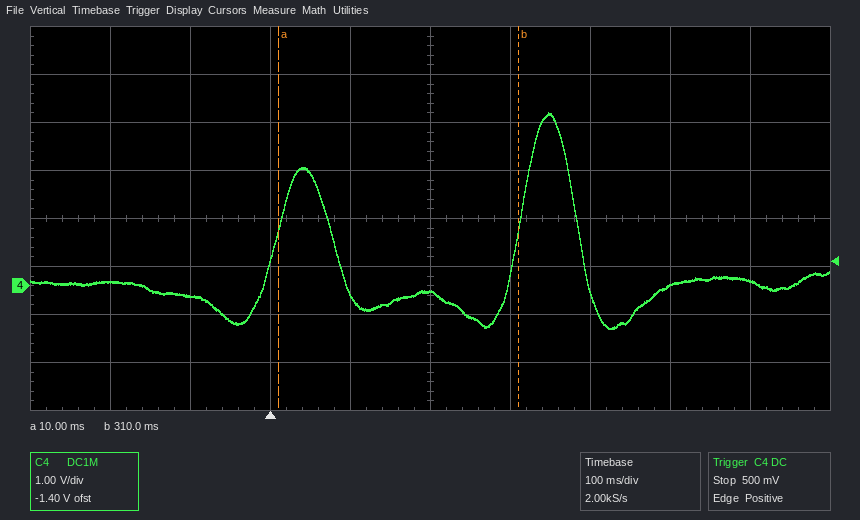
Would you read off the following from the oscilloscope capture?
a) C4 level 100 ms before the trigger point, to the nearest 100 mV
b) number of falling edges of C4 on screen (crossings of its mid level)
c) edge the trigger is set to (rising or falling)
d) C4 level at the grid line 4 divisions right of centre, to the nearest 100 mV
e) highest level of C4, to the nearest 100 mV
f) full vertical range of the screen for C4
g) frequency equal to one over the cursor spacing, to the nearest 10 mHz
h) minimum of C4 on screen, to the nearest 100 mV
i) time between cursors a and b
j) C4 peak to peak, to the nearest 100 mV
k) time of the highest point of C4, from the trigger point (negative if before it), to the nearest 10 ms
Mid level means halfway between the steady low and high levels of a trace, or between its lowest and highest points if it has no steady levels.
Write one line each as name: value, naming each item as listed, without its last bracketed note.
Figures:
C4 level 100 ms before the trigger point, to the nearest 100 mV: -200 mV
number of falling edges of C4 on screen: 2
edge the trigger is set to: rising
C4 level at the grid line 4 divisions right of centre, to the nearest 100 mV: 100 mV
highest level of C4, to the nearest 100 mV: 3.6 V
full vertical range of the screen for C4: 8 V
frequency equal to one over the cursor spacing, to the nearest 10 mHz: 3.33 Hz
minimum of C4 on screen, to the nearest 100 mV: -900 mV
time between cursors a and b: 300 ms
C4 peak to peak, to the nearest 100 mV: 4.5 V
time of the highest point of C4, from the trigger point (negative if before it), to the nearest 10 ms: +350 ms
